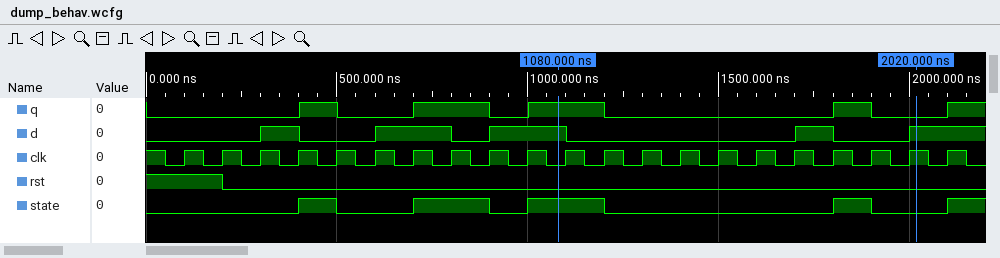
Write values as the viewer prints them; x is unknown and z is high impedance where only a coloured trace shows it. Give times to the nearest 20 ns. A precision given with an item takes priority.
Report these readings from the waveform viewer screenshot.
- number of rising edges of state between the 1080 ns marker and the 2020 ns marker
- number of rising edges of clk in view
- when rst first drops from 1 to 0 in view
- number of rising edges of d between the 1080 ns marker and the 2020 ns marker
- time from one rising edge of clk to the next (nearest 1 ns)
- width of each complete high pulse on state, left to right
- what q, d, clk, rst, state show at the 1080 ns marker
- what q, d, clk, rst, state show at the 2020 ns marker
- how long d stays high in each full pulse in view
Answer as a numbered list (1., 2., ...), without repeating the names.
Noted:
1. 1
2. 21
3. 200 ns
4. 2
5. 100 ns
6. 100 ns, 200 ns, 200 ns, 100 ns
7. q=1, d=1, clk=0, rst=0, state=1
8. q=0, d=1, clk=1, rst=0, state=0
9. 100 ns, 200 ns, 200 ns, 100 ns
